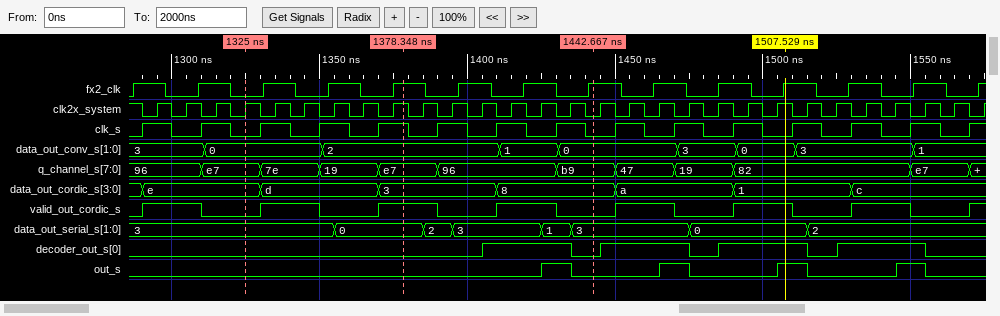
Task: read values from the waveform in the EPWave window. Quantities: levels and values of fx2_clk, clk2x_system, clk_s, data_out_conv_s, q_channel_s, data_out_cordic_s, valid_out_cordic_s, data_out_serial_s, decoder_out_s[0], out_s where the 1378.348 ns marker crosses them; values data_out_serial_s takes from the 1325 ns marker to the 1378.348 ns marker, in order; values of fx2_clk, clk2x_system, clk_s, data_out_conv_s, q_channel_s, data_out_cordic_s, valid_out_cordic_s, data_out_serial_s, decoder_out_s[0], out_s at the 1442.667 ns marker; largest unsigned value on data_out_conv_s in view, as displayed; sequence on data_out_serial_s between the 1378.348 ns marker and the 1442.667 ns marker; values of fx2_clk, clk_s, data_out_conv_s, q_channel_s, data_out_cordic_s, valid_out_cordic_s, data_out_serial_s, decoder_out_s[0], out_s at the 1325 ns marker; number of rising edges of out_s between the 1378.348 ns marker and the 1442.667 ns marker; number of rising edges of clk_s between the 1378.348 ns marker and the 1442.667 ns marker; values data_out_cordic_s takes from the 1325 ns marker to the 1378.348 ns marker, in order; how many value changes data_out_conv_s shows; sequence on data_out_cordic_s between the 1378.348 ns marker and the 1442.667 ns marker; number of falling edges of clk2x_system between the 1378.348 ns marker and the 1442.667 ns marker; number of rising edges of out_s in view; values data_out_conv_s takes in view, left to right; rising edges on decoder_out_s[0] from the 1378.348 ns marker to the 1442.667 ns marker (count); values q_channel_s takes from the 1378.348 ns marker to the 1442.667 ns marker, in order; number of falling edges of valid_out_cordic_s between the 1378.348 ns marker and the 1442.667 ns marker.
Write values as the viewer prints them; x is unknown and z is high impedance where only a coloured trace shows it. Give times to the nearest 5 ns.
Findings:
fx2_clk=1, clk2x_system=1, clk_s=1, data_out_conv_s=2, q_channel_s=e7, data_out_cordic_s=3, valid_out_cordic_s=1, data_out_serial_s=0, decoder_out_s[0]=0, out_s=0
3, 0
fx2_clk=1, clk2x_system=0, clk_s=0, data_out_conv_s=0, q_channel_s=b9, data_out_cordic_s=8, valid_out_cordic_s=0, data_out_serial_s=3, decoder_out_s[0]=0, out_s=0
3
0, 2, 3, 1, 3
fx2_clk=0, clk_s=0, data_out_conv_s=0, q_channel_s=e7, data_out_cordic_s=e, valid_out_cordic_s=0, data_out_serial_s=3, decoder_out_s[0]=0, out_s=0
1
3
e, d, 3
8
3, 8
7
4
3, 0, 2, 1, 0, 3, 0, 3, 1
1
e7, 96, b9
2
